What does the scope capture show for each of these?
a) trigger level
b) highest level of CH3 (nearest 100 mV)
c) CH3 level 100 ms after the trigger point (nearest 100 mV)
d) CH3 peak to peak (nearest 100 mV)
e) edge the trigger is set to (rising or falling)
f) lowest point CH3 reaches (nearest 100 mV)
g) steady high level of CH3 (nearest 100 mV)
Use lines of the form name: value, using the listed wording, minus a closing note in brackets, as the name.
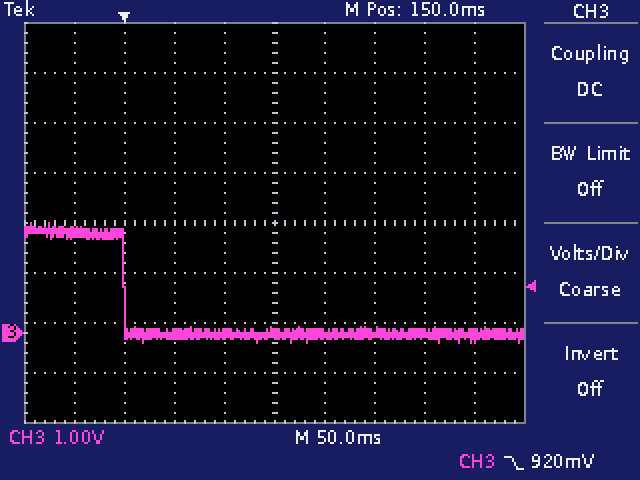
trigger level: 920 mV
highest level of CH3: 2.2 V
CH3 level 100 ms after the trigger point: 0.0 V
CH3 peak to peak: 2.4 V
edge the trigger is set to: falling
lowest point CH3 reaches: -200 mV
steady high level of CH3: 2.0 V
